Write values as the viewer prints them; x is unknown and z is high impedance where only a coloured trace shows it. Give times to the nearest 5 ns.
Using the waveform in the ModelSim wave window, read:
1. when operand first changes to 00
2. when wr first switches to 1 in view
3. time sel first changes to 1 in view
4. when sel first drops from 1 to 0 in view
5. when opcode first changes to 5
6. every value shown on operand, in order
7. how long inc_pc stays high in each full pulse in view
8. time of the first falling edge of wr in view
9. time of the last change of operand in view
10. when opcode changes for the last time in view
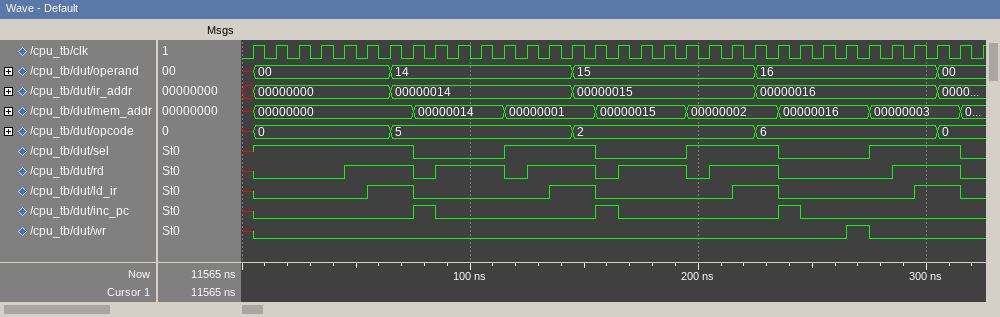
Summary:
5 ns
265 ns
5 ns
75 ns
65 ns
x, 00, 14, 15, 16, 00
10 ns, 10 ns, 10 ns
275 ns
305 ns
305 ns
